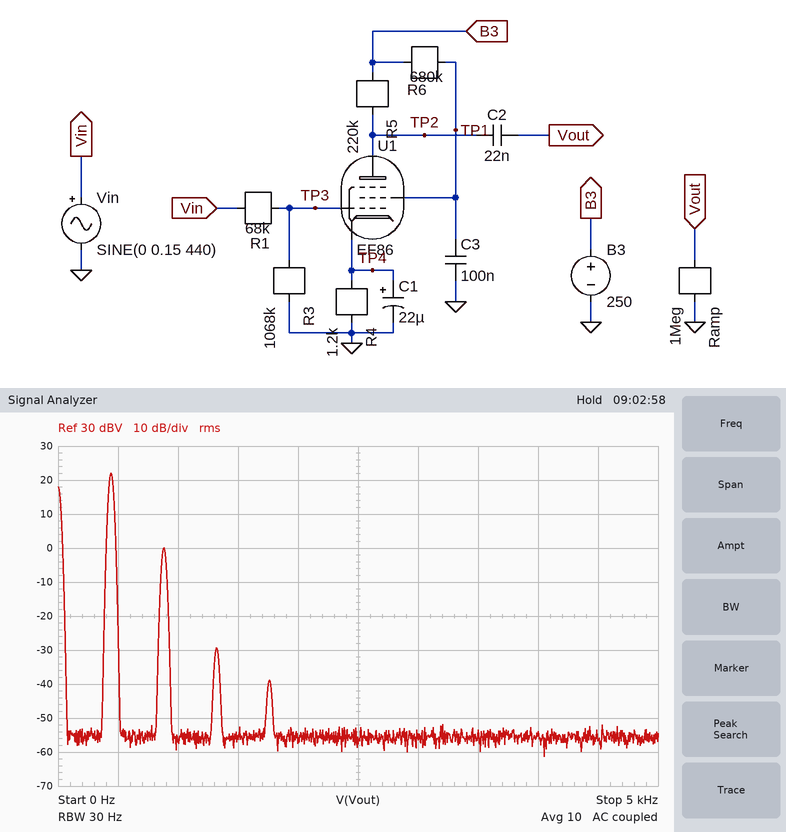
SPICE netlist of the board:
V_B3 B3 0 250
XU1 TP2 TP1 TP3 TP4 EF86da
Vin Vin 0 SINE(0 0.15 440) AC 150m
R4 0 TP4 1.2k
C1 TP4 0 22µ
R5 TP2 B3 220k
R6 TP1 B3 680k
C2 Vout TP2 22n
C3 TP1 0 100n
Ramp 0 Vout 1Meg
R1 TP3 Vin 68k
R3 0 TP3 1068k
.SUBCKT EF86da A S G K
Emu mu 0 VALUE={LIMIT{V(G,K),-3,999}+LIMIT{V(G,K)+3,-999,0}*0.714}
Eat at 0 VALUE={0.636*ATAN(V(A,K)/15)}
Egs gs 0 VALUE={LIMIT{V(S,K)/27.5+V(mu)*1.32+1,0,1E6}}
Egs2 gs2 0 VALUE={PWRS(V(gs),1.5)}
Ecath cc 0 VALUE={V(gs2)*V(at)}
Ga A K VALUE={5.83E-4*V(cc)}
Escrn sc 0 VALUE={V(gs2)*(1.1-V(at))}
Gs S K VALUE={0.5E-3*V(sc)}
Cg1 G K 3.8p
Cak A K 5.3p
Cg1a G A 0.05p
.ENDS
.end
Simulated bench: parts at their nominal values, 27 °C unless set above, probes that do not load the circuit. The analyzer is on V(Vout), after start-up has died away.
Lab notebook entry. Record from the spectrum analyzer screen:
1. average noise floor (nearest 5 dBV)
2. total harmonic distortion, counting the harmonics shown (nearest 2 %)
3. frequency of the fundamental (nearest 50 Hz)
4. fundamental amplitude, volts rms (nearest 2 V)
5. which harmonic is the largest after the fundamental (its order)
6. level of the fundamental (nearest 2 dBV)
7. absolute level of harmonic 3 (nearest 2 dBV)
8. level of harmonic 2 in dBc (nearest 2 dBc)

-55 dBV
8 %
450 Hz
12 V
2
22 dBV
-30 dBV
-22 dBc
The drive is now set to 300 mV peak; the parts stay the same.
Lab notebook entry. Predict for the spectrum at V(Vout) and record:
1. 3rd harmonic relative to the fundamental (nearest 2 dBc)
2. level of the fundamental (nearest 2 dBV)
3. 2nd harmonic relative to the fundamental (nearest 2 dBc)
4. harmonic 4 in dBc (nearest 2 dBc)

-38 dBc
28 dBV
-18 dBc
-46 dBc
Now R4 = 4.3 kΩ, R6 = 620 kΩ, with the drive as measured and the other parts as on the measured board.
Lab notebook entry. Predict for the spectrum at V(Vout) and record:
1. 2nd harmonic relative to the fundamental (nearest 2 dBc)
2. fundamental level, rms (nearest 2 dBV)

-34 dBc
22 dBV
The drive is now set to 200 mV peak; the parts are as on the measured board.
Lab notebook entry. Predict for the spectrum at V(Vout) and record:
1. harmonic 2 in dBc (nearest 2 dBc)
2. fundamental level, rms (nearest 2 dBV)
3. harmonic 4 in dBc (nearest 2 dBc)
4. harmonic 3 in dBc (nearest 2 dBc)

-20 dBc
24 dBV
-54 dBc
-46 dBc
